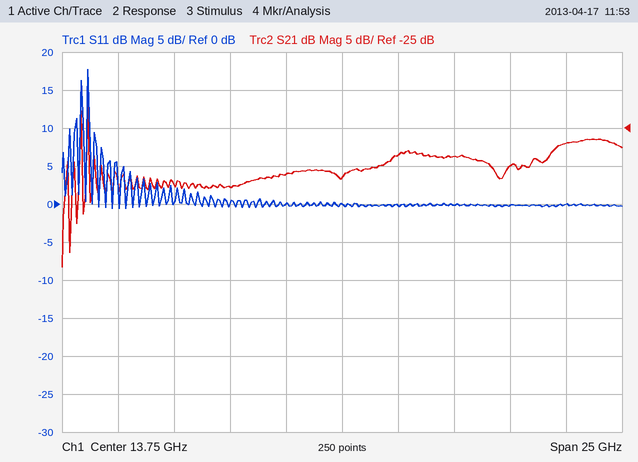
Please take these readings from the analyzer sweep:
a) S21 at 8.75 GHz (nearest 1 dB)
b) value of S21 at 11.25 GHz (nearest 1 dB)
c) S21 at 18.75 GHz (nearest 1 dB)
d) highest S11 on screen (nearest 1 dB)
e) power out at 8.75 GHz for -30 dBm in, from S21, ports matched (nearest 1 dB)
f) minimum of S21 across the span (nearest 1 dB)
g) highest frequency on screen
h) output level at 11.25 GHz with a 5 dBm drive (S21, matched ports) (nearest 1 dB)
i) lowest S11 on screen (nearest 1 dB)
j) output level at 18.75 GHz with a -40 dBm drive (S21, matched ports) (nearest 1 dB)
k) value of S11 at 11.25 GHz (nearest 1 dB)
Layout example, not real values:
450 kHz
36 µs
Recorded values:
-33 dB
-31 dB
-29 dB
18 dB
-63 dBm
-43 dB
26.25 GHz
-26 dBm
-1 dB
-69 dBm
0 dB
